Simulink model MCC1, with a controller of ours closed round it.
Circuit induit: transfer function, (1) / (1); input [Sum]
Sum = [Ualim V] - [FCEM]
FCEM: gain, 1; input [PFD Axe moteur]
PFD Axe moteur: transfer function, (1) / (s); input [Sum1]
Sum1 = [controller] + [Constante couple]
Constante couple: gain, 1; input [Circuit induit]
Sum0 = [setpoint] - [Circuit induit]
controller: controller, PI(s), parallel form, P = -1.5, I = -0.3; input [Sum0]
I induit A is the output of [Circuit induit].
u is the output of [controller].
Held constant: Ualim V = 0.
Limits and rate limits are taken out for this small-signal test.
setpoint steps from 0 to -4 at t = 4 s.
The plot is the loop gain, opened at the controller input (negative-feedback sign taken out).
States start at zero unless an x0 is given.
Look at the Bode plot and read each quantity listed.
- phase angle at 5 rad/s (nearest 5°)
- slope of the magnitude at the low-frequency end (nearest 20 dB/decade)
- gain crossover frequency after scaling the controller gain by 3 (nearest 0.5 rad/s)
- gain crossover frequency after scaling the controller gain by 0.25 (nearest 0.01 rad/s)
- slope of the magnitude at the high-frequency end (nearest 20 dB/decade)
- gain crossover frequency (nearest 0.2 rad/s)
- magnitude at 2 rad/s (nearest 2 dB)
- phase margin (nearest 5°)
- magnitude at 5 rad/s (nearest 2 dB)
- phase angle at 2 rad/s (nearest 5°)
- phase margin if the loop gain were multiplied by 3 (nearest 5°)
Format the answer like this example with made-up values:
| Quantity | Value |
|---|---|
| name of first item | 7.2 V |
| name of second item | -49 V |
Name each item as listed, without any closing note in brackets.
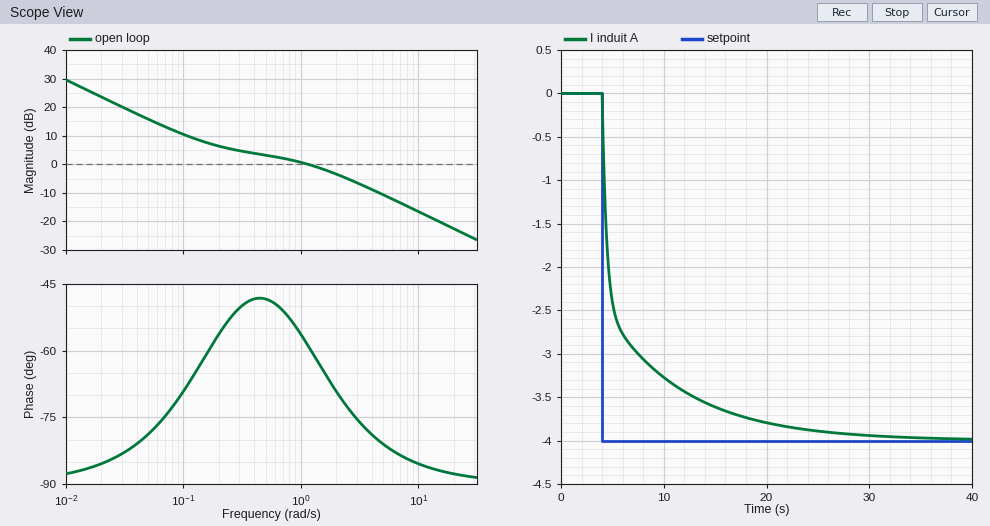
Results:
| Quantity | Value |
|---|---|
| phase angle at 5 rad/s | -80° |
| slope of the magnitude at the low-frequency end | -20 dB/decade |
| gain crossover frequency after scaling the controller gain by 3 | 4.5 rad/s |
| gain crossover frequency after scaling the controller gain by 0.25 | 0.08 rad/s |
| slope of the magnitude at the high-frequency end | -20 dB/decade |
| gain crossover frequency | 1.2 rad/s |
| magnitude at 2 rad/s | -4 dB |
| phase margin | 120° |
| magnitude at 5 rad/s | -10 dB |
| phase angle at 2 rad/s | -70° |
| phase margin if the loop gain were multiplied by 3 | 100° |
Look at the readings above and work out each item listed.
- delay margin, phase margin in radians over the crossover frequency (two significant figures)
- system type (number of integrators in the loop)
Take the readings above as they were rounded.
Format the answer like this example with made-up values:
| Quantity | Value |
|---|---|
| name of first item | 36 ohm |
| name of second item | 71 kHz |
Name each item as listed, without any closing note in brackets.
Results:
| Quantity | Value |
|---|---|
| delay margin, phase margin in radians over the crossover frequency | 1.7 s |
| system type | 1 |
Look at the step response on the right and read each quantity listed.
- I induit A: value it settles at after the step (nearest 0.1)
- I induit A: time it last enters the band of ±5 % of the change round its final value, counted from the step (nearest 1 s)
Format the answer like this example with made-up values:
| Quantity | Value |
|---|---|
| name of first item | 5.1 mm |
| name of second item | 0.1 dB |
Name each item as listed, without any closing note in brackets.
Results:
| Quantity | Value |
|---|---|
| I induit A: value it settles at after the step | -4.0 |
| I induit A: time it last enters the band of ±5 % of the change round its final value, counted from the step | 16 s |
